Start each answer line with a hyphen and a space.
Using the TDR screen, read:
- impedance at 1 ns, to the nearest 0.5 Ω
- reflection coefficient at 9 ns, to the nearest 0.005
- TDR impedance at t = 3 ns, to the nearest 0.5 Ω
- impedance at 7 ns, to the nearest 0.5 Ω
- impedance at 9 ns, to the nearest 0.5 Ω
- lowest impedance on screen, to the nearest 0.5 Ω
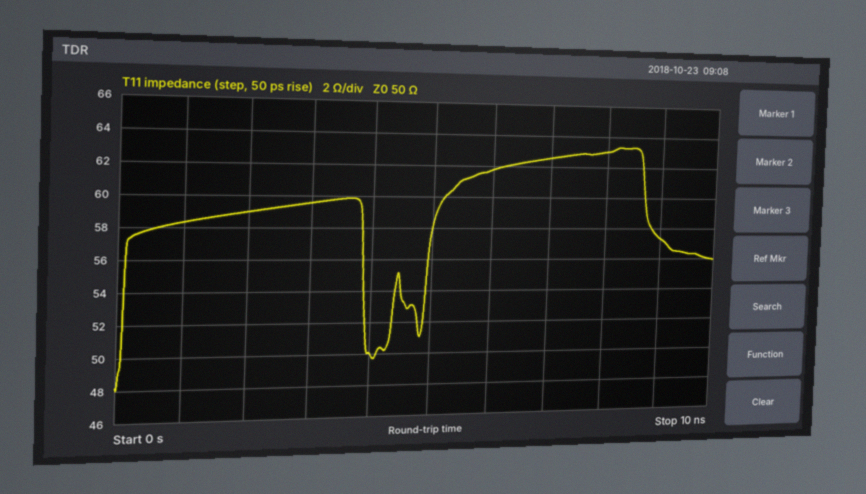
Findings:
- 58.5 Ω
- +0.070
- 59.5 Ω
- 62.5 Ω
- 57.5 Ω
- 48.0 Ω
